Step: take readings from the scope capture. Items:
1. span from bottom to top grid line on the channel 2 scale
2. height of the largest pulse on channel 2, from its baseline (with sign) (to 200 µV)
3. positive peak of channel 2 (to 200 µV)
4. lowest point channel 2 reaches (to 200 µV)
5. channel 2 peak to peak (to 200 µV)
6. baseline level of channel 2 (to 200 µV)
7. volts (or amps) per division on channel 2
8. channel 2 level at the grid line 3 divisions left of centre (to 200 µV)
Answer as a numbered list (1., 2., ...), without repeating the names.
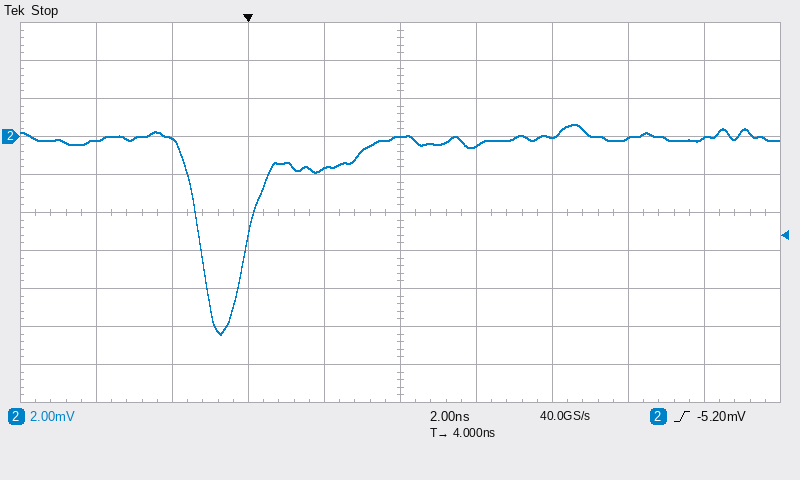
1. 20 mV
2. -10.2 mV
3. 600 µV
4. -10.4 mV
5. 11.0 mV
6. -200 µV
7. 2 mV
8. -200 µV
